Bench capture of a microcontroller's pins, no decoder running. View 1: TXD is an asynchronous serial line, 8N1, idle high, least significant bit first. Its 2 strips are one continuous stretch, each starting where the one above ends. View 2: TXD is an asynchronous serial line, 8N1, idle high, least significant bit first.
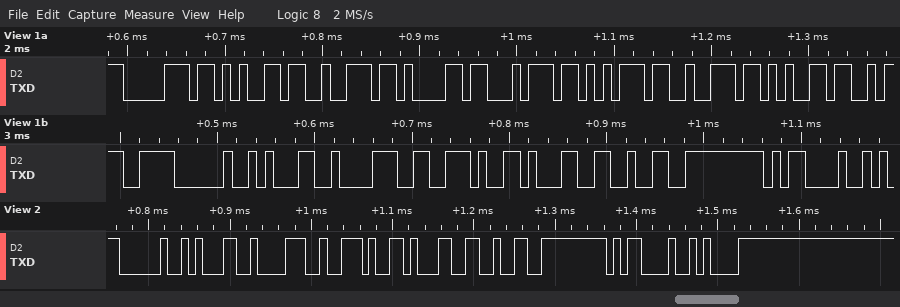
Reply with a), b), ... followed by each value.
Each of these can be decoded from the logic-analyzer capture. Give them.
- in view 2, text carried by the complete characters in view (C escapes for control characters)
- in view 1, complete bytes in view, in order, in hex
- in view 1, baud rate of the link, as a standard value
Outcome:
a) " 18.12\r\n"
b) 70 65 72 61 74 75 72 65 3A 20 31 38 2E 31 32 0D
c) 115200 baud
